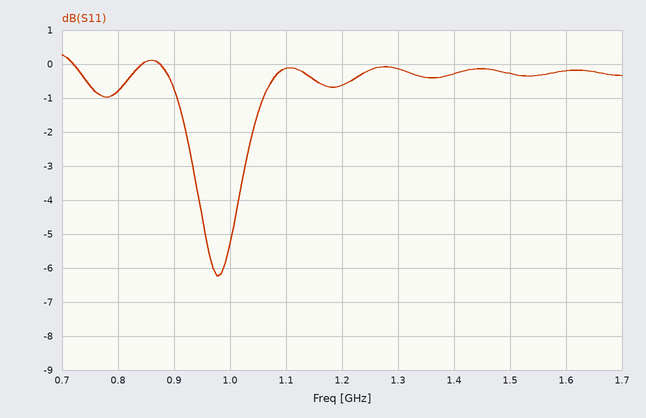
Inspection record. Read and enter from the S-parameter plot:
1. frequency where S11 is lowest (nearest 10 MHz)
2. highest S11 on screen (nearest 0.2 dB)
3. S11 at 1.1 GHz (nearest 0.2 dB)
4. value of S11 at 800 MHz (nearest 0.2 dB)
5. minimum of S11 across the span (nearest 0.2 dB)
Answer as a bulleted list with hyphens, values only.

- 980 MHz
- 0.2 dB
- -0.2 dB
- -0.8 dB
- -6.2 dB
